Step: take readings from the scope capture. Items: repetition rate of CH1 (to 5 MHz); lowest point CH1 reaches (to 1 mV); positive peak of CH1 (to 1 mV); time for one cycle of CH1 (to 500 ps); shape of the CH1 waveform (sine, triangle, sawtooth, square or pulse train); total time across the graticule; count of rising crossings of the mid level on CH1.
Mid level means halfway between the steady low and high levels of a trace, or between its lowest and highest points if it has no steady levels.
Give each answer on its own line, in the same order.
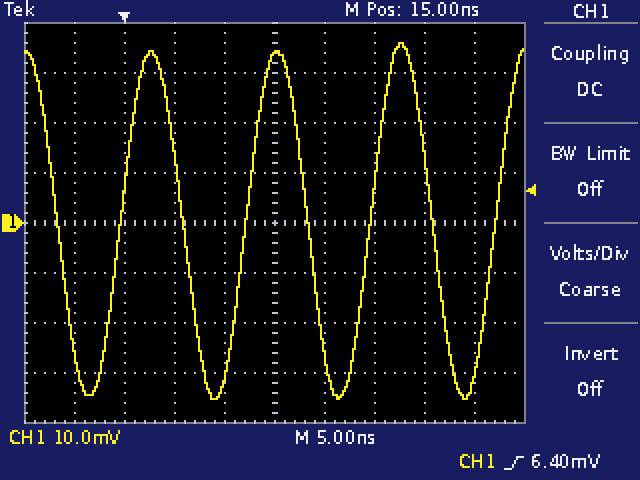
80 MHz
-35 mV
36 mV
12.5 ns
sine
50 ns
4
